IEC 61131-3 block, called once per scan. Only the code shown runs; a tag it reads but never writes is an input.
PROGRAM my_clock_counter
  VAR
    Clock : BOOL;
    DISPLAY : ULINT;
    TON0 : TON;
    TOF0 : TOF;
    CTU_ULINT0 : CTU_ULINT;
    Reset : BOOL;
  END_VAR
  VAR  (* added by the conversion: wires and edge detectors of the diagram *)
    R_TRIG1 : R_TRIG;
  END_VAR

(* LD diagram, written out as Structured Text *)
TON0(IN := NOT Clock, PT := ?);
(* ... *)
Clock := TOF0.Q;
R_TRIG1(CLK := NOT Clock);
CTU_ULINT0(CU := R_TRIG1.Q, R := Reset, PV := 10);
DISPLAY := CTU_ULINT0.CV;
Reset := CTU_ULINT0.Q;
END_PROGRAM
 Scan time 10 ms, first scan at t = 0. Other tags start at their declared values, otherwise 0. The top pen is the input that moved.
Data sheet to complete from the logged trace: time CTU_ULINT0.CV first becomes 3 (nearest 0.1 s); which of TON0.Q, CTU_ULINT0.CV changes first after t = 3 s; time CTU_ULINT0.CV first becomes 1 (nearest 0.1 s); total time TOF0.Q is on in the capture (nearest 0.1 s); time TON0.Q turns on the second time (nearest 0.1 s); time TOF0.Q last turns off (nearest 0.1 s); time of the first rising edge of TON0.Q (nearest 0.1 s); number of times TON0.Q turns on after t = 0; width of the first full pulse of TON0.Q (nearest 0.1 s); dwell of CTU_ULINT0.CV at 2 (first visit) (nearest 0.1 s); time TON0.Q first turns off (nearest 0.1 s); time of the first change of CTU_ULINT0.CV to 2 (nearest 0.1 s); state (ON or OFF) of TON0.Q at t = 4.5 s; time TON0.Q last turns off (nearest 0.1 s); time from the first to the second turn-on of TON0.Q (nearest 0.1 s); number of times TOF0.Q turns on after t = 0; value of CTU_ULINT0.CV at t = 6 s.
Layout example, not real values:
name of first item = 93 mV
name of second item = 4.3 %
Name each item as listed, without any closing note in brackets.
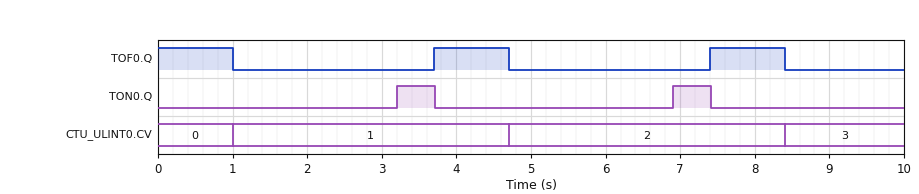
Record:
time CTU_ULINT0.CV first becomes 3 = 8.4 s
which of TON0.Q, CTU_ULINT0.CV changes first after t = 3 s = TON0.Q
time CTU_ULINT0.CV first becomes 1 = 1.0 s
total time TOF0.Q is on in the capture = 3.0 s
time TON0.Q turns on the second time = 6.9 s
time TOF0.Q last turns off = 8.4 s
time of the first rising edge of TON0.Q = 3.2 s
number of times TON0.Q turns on after t = 0 = 2
width of the first full pulse of TON0.Q = 0.5 s
dwell of CTU_ULINT0.CV at 2 (first visit) = 3.7 s
time TON0.Q first turns off = 3.7 s
time of the first change of CTU_ULINT0.CV to 2 = 4.7 s
state (ON or OFF) of TON0.Q at t = 4.5 s = OFF
time TON0.Q last turns off = 7.4 s
time from the first to the second turn-on of TON0.Q = 3.7 s
number of times TOF0.Q turns on after t = 0 = 2
value of CTU_ULINT0.CV at t = 6 s = 2
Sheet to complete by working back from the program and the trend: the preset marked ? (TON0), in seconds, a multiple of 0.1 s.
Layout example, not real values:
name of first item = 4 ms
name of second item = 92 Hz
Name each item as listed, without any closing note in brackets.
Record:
the preset marked ? (TON0), in seconds, a multiple of 0.1 s = 2.2 s
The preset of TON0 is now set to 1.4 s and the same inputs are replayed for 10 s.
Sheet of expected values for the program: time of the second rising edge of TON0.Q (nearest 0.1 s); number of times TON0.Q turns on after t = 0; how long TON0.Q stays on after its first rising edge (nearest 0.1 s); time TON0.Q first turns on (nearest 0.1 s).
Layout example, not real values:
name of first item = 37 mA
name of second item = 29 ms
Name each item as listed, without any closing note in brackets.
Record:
time of the second rising edge of TON0.Q = 6.1 s
number of times TON0.Q turns on after t = 0 = 3
how long TON0.Q stays on after its first rising edge = 1.3 s
time TON0.Q first turns on = 2.4 s
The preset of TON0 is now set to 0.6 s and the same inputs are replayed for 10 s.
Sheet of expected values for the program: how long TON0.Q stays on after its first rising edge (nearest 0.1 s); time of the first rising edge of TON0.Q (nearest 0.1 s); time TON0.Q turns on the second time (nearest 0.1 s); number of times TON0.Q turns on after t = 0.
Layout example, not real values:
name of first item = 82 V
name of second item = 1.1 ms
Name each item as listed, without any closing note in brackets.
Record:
how long TON0.Q stays on after its first rising edge = 2.1 s
time of the first rising edge of TON0.Q = 1.6 s
time TON0.Q turns on the second time = 5.3 s
number of times TON0.Q turns on after t = 0 = 3
